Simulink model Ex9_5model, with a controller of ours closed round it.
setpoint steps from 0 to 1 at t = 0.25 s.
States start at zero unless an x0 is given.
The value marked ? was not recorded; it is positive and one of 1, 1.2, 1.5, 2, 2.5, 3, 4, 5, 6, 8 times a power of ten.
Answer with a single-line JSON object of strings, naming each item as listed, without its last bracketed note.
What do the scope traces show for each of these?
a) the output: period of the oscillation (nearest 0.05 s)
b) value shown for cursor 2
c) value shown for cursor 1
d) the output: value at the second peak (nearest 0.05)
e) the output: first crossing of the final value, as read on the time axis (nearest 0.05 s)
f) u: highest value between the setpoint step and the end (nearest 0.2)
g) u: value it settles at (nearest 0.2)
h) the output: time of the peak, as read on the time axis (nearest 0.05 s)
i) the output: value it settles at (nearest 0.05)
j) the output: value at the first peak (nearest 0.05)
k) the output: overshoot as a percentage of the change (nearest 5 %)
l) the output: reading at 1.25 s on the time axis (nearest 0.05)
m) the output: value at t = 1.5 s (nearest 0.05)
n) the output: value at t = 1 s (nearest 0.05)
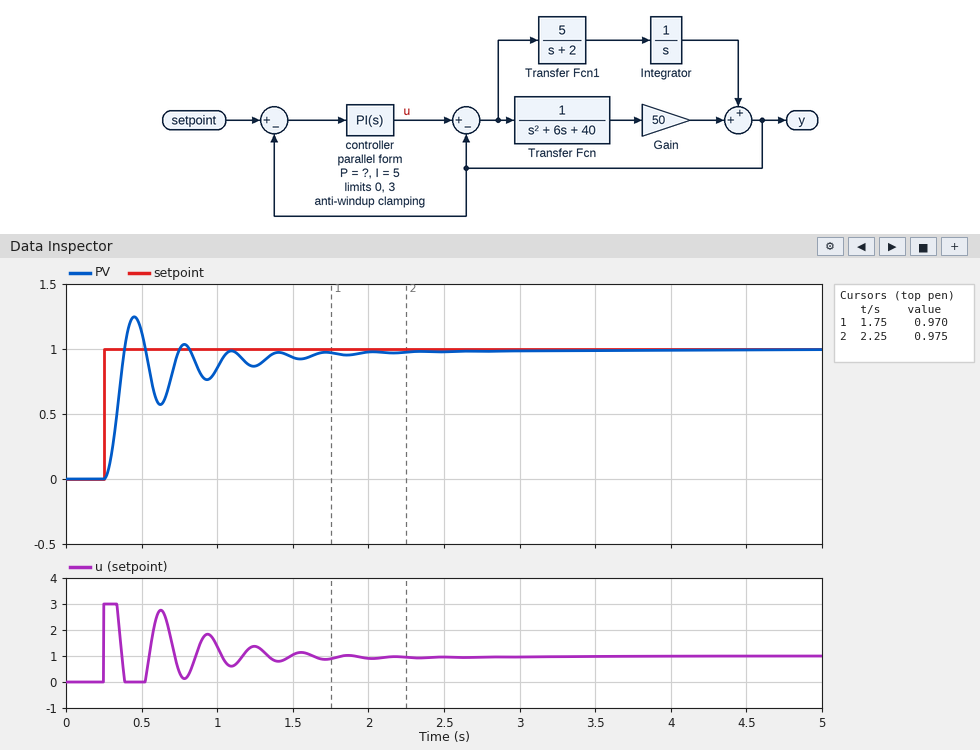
{"the output: period of the oscillation": "0.35 s", "value shown for cursor 2": "0.975", "value shown for cursor 1": "0.970", "the output: value at the second peak": "1.05", "the output: first crossing of the final value, as read on the time axis": "0.40 s", "u: highest value between the setpoint step and the end": "3.0", "u: value it settles at": "1.0", "the output: time of the peak, as read on the time axis": "0.45 s", "the output: value it settles at": "1.00", "the output: value at the first peak": "1.25", "the output: overshoot as a percentage of the change": "25 %", "the output: reading at 1.25 s on the time axis": "0.85", "the output: value at t = 1.5 s": "0.95", "the output: value at t = 1 s": "0.85"}
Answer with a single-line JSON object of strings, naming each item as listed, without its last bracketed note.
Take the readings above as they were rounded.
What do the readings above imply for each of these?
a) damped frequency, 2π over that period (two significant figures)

{"damped frequency, 2π over that period": "18 rad/s"}
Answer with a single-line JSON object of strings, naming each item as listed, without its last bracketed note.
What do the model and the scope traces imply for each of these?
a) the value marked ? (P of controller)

{"the value marked ?": "6"}
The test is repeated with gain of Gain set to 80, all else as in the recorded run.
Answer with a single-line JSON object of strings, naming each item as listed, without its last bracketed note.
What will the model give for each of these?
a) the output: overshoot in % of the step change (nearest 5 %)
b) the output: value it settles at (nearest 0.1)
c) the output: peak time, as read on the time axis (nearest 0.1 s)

{"the output: overshoot in % of the step change": "35 %", "the output: value it settles at": "1.0", "the output: peak time, as read on the time axis": "0.4 s"}
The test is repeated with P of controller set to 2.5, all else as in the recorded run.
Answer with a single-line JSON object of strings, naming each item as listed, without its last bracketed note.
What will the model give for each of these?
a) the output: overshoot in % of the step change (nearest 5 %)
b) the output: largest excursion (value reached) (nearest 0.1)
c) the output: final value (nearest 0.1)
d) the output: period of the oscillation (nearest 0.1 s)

{"the output: overshoot in % of the step change": "10 %", "the output: largest excursion (value reached)": "1.1", "the output: final value": "1.0", "the output: period of the oscillation": "0.4 s"}
